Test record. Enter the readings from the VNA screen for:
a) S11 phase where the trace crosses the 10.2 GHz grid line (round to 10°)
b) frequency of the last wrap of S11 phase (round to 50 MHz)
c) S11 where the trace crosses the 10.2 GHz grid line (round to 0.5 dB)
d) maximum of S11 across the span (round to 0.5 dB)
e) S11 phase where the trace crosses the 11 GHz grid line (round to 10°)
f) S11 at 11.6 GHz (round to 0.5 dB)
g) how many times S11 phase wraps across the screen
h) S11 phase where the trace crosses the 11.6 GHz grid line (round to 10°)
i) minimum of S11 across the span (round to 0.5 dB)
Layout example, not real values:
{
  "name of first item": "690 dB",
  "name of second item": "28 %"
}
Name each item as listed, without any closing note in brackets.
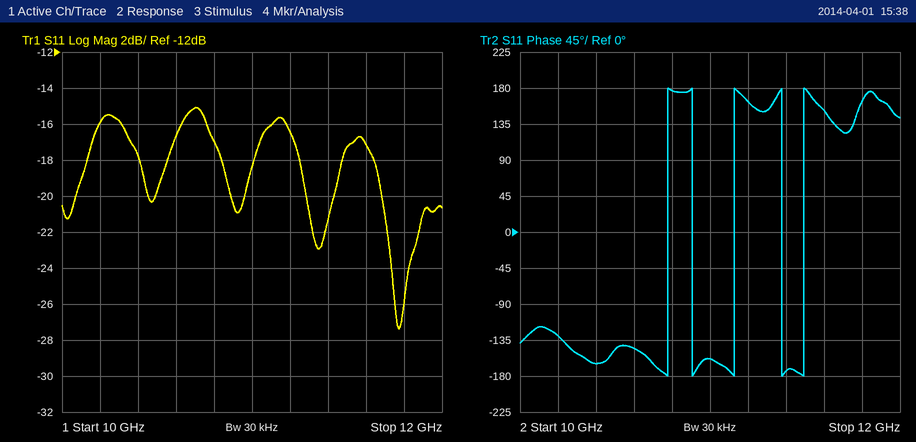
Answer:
{
  "S11 phase where the trace crosses the 10.2 GHz grid line": "-130°",
  "frequency of the last wrap of S11 phase": "11.50 GHz",
  "S11 where the trace crosses the 10.2 GHz grid line": "-16.0 dB",
  "maximum of S11 across the span": "-15.0 dB",
  "S11 phase where the trace crosses the 11 GHz grid line": "-160°",
  "S11 at 11.6 GHz": "-17.0 dB",
  "how many times S11 phase wraps across the screen": "5",
  "S11 phase where the trace crosses the 11.6 GHz grid line": "150°",
  "minimum of S11 across the span": "-27.5 dB"
}
